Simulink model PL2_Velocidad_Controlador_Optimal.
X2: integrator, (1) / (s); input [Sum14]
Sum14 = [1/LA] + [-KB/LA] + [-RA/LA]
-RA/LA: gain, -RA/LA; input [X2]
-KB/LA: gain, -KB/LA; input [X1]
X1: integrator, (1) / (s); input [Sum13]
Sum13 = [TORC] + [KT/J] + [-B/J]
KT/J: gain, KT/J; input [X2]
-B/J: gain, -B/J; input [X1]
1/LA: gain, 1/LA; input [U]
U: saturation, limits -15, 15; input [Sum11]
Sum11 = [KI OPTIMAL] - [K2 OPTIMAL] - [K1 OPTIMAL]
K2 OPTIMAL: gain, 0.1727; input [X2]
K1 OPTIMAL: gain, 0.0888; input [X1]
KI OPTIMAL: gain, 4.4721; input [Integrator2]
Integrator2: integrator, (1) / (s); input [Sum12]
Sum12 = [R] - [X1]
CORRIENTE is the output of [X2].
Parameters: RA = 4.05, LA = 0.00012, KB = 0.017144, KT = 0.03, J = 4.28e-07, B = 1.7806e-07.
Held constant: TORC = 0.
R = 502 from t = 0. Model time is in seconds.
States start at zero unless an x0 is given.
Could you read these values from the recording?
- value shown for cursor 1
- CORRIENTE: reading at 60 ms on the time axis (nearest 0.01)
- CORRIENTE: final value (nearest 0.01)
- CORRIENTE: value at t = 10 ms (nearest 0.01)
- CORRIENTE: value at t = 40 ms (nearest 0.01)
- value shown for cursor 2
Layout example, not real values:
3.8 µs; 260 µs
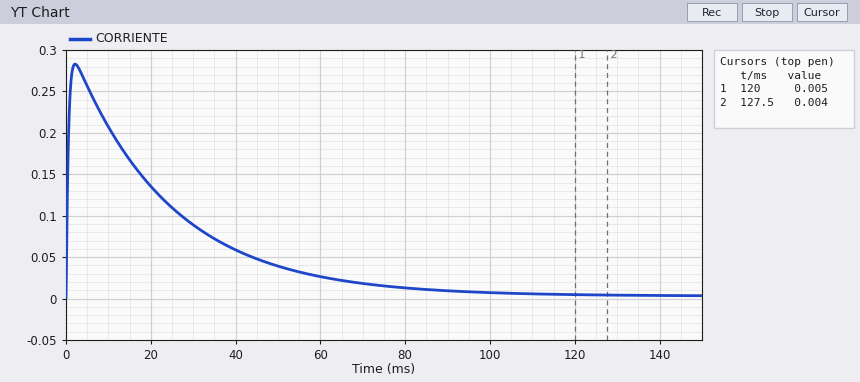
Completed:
0.005; 0.03; 0.00; 0.21; 0.06; 0.004
